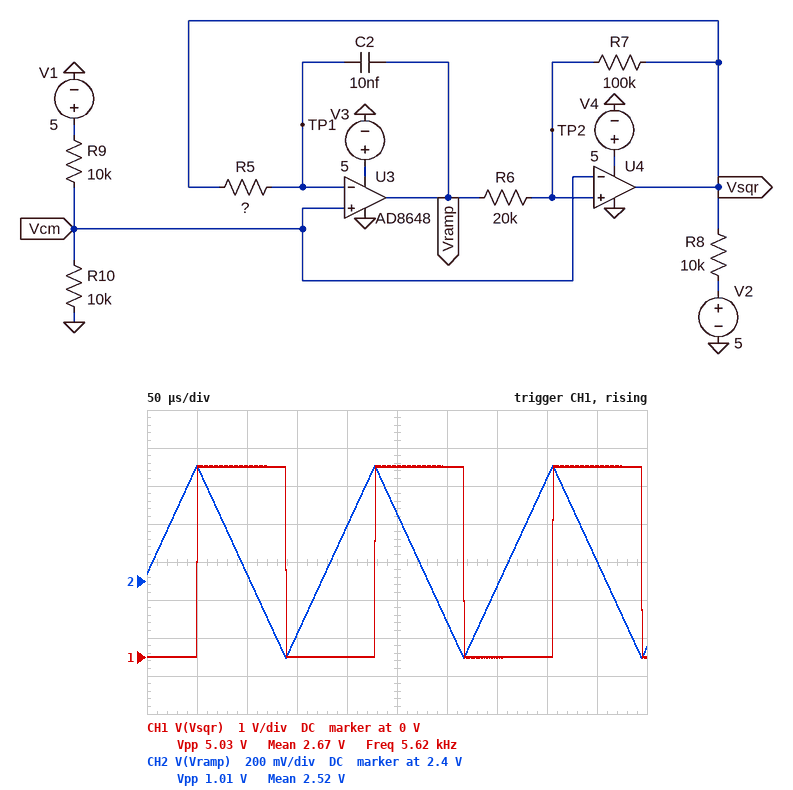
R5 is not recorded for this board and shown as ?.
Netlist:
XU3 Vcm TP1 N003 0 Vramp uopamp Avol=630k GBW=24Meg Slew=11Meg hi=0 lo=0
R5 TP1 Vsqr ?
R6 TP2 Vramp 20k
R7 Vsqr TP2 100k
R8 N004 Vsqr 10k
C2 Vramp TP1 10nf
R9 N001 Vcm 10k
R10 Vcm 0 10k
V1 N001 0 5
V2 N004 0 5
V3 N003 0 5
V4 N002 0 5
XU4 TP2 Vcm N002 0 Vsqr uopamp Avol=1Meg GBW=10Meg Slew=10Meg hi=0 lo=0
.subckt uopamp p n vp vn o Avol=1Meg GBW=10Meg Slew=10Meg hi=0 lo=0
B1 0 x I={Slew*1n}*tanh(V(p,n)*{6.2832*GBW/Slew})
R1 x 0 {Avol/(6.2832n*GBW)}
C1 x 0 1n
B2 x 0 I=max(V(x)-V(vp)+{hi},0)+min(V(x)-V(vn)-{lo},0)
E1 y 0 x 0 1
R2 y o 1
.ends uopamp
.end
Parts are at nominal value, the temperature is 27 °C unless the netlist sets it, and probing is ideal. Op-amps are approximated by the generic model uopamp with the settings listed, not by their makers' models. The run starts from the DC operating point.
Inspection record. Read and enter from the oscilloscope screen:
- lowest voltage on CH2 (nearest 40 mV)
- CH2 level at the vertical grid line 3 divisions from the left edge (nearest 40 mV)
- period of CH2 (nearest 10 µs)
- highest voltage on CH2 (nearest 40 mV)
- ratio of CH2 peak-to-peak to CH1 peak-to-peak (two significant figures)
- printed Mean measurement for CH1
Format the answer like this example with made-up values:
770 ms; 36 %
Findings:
2.00 V; 2.12 V; 180 µs; 3.00 V; 0.20; 2.67 V
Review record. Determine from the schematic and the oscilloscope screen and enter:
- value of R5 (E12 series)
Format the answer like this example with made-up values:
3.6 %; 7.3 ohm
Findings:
22 kΩ
